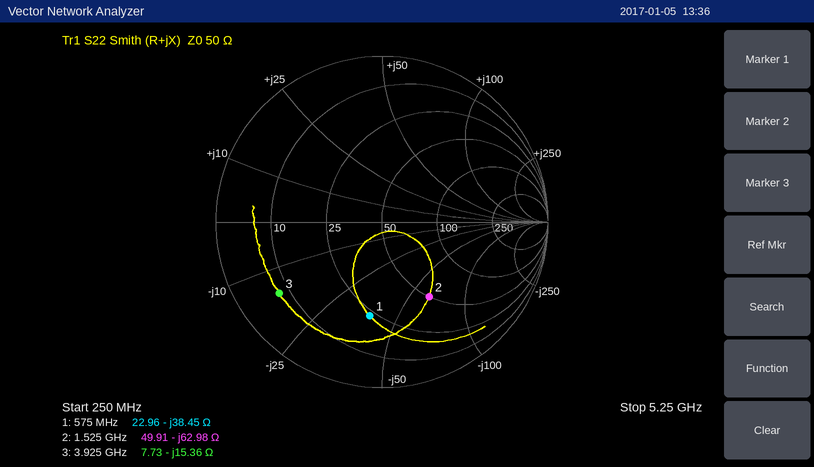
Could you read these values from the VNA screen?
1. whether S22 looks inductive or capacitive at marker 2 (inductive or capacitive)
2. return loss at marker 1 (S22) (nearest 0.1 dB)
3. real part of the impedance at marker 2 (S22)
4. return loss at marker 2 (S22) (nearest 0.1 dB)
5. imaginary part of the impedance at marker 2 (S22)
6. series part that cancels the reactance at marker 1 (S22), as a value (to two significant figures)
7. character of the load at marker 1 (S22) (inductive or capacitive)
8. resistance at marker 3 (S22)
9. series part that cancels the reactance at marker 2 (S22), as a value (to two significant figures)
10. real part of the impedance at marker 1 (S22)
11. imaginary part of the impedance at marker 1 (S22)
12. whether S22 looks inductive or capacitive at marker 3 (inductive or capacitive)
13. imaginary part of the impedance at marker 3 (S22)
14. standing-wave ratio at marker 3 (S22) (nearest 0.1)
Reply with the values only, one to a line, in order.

capacitive
4.9 dB
49.91 Ω
5.5 dB
-62.98 Ω
11 nH
capacitive
7.73 Ω
6.6 nH
22.96 Ω
-38.45 Ω
capacitive
-15.36 Ω
7.1
